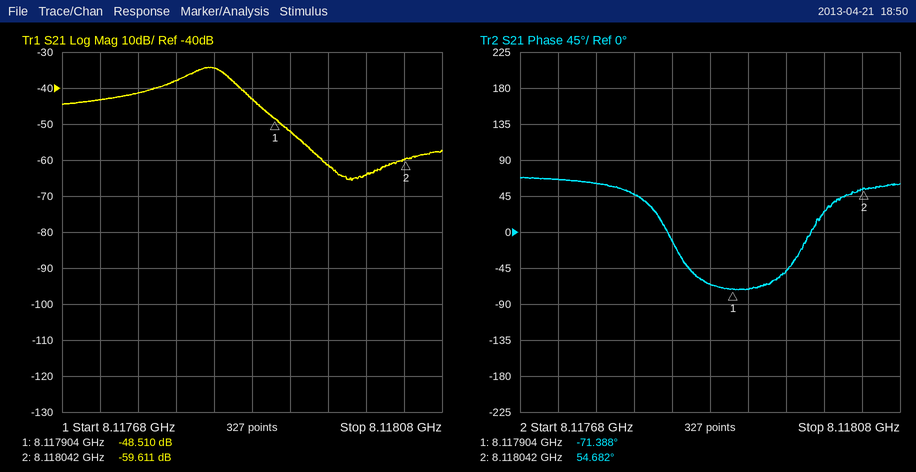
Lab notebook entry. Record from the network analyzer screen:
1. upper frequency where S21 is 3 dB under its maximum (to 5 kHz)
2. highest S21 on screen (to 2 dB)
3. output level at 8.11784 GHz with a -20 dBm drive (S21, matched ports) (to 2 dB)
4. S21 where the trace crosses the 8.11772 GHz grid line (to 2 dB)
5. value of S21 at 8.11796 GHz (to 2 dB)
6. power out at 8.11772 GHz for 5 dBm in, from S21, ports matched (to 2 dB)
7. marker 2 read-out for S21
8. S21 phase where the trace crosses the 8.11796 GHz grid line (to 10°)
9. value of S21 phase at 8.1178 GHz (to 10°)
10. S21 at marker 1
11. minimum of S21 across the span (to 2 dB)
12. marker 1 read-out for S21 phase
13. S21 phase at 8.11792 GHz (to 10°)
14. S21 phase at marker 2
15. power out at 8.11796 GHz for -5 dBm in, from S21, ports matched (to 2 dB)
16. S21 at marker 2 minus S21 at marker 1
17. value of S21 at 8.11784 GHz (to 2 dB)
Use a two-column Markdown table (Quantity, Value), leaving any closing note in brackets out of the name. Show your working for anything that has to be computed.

| Quantity | Value |
|---|---|
| upper frequency where S21 is 3 dB under its maximum | 8.117855 GHz |
| highest S21 on screen | -34 dB |
| output level at 8.11784 GHz with a -20 dBm drive (S21, matched ports) | -20 dBm + (-34 dB) = -54 dBm |
| S21 where the trace crosses the 8.11772 GHz grid line | -44 dB |
| value of S21 at 8.11796 GHz | -62 dB |
| power out at 8.11772 GHz for 5 dBm in, from S21, ports matched | 5 dBm + (-44 dB) = -38 dBm |
| marker 2 read-out for S21 | -59.611 dB |
| S21 phase where the trace crosses the 8.11796 GHz grid line | -50° |
| value of S21 phase at 8.1178 GHz | 50° |
| S21 at marker 1 | -48.510 dB |
| minimum of S21 across the span | -66 dB |
| marker 1 read-out for S21 phase | -71.388° |
| S21 phase at 8.11792 GHz | -70° |
| S21 phase at marker 2 | 54.682° |
| power out at 8.11796 GHz for -5 dBm in, from S21, ports matched | -5 dBm + (-62 dB) = -66 dBm |
| S21 at marker 2 minus S21 at marker 1 | -59.611 − (-48.51) = -11.101 dB |
| value of S21 at 8.11784 GHz | -34 dB |
